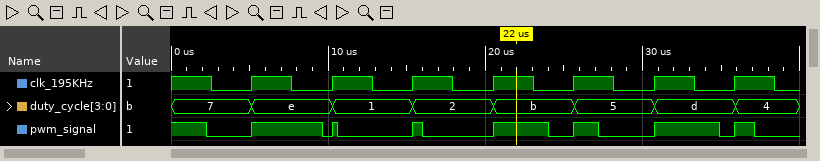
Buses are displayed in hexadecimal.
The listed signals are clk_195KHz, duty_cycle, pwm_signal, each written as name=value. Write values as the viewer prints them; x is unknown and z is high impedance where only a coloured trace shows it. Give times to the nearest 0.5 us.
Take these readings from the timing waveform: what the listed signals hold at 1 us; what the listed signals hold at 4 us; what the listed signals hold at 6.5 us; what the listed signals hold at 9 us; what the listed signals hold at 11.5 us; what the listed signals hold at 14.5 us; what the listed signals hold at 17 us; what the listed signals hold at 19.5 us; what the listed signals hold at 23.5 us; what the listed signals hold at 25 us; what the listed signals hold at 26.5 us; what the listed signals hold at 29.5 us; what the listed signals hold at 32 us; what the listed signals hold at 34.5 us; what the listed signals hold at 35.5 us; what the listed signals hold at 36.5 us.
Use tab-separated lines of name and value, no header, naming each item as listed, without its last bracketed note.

what the listed signals hold at 1 us	clk_195KHz=1, duty_cycle=7, pwm_signal=1
what the listed signals hold at 4 us	clk_195KHz=0, duty_cycle=7, pwm_signal=0
what the listed signals hold at 6.5 us	clk_195KHz=1, duty_cycle=e, pwm_signal=1
what the listed signals hold at 9 us	clk_195KHz=0, duty_cycle=e, pwm_signal=1
what the listed signals hold at 11.5 us	clk_195KHz=1, duty_cycle=1, pwm_signal=0
what the listed signals hold at 14.5 us	clk_195KHz=0, duty_cycle=1, pwm_signal=0
what the listed signals hold at 17 us	clk_195KHz=1, duty_cycle=2, pwm_signal=0
what the listed signals hold at 19.5 us	clk_195KHz=0, duty_cycle=2, pwm_signal=0
what the listed signals hold at 23.5 us	clk_195KHz=0, duty_cycle=b, pwm_signal=1
what the listed signals hold at 25 us	clk_195KHz=0, duty_cycle=b, pwm_signal=0
what the listed signals hold at 26.5 us	clk_195KHz=1, duty_cycle=5, pwm_signal=1
what the listed signals hold at 29.5 us	clk_195KHz=0, duty_cycle=5, pwm_signal=0
what the listed signals hold at 32 us	clk_195KHz=1, duty_cycle=d, pwm_signal=1
what the listed signals hold at 34.5 us	clk_195KHz=0, duty_cycle=d, pwm_signal=1
what the listed signals hold at 35.5 us	clk_195KHz=0, duty_cycle=d, pwm_signal=0
what the listed signals hold at 36.5 us	clk_195KHz=1, duty_cycle=4, pwm_signal=1
